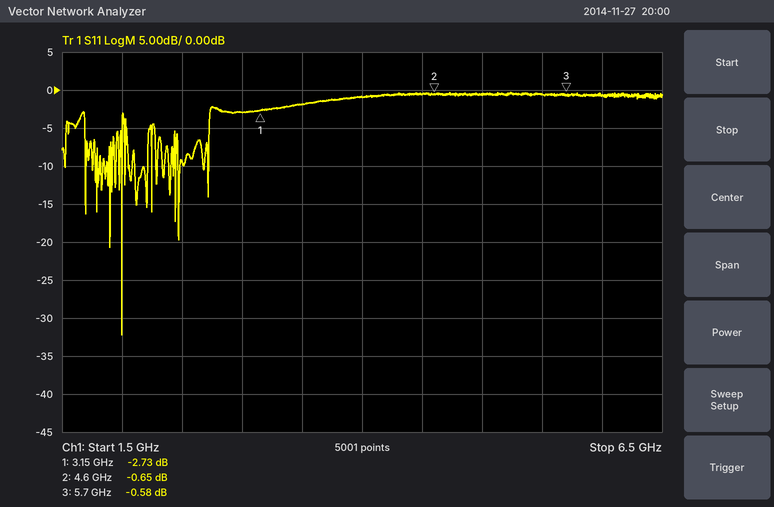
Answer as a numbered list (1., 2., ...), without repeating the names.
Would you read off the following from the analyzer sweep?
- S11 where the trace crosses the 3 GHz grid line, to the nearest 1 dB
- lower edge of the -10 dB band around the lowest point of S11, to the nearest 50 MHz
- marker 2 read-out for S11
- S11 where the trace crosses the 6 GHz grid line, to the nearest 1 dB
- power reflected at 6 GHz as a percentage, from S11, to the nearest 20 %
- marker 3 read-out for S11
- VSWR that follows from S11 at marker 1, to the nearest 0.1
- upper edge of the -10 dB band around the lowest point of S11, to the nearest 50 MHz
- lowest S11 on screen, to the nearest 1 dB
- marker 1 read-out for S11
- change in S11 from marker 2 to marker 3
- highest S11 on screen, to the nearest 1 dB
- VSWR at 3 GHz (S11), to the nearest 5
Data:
1. -3 dB
2. 2.00 GHz
3. -0.65 dB
4. -1 dB
5. 80 %
6. -0.58 dB
7. 6.4
8. 2.00 GHz
9. -32 dB
10. -2.73 dB
11. 0.07 dB
12. 0 dB
13. 5
